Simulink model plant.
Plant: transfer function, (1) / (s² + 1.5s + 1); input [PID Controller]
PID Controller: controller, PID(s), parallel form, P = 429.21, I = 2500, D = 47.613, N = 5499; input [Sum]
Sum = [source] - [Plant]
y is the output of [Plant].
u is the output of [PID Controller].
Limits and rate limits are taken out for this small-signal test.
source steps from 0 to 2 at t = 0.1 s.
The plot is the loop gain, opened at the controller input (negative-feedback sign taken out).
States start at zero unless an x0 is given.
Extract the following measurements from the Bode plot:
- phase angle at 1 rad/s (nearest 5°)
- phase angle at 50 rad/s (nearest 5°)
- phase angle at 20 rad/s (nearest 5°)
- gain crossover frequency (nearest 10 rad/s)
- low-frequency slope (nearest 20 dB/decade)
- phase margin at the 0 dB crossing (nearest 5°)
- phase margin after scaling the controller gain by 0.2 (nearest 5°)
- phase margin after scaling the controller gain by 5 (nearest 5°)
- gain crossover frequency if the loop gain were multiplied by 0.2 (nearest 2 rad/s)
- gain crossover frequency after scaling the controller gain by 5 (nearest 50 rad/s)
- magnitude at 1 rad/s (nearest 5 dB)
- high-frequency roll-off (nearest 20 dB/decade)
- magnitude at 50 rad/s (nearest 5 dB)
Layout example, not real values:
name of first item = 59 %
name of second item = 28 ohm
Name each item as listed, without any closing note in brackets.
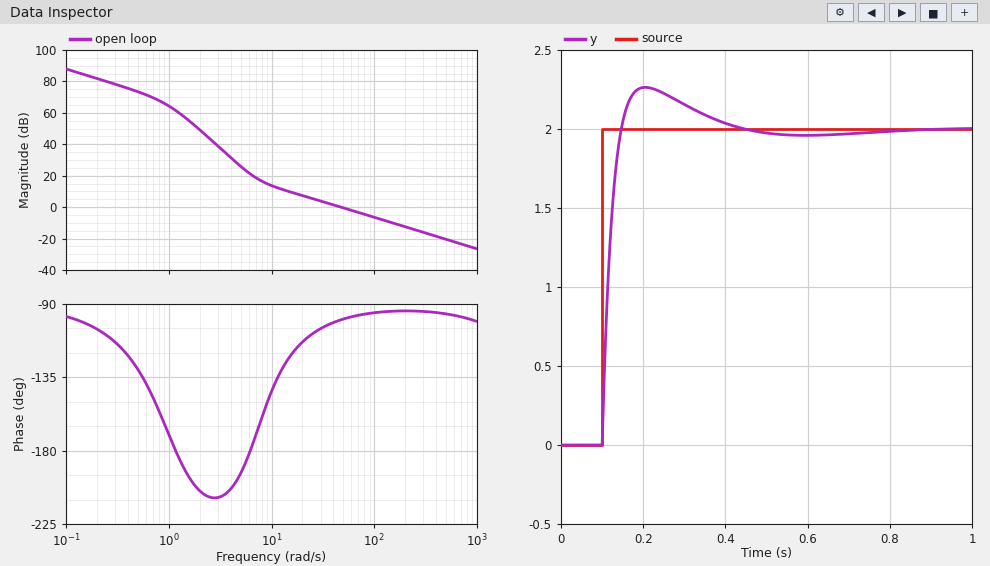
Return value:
phase angle at 1 rad/s = -170°
phase angle at 50 rad/s = -100°
phase angle at 20 rad/s = -115°
gain crossover frequency = 50 rad/s
low-frequency slope = -20 dB/decade
phase margin at the 0 dB crossing = 80°
phase margin after scaling the controller gain by 0.2 = 35°
phase margin after scaling the controller gain by 5 = 85°
gain crossover frequency if the loop gain were multiplied by 0.2 = 10 rad/s
gain crossover frequency after scaling the controller gain by 5 = 250 rad/s
magnitude at 1 rad/s = 65 dB
high-frequency roll-off = -20 dB/decade
magnitude at 50 rad/s = 0 dB
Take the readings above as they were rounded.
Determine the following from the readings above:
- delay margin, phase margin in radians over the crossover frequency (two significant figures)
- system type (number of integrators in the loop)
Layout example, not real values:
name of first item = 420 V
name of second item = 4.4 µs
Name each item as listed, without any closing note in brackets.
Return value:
delay margin, phase margin in radians over the crossover frequency = 0.028 s
system type = 1
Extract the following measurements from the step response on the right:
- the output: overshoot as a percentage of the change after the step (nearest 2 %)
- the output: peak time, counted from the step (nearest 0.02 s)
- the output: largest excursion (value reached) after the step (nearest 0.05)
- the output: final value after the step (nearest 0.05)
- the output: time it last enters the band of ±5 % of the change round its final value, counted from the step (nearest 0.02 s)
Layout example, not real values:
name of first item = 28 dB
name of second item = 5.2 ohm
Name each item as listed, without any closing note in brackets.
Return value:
the output: overshoot as a percentage of the change after the step = 14 %
the output: peak time, counted from the step = 0.10 s
the output: largest excursion (value reached) after the step = 2.25
the output: final value after the step = 2.00
the output: time it last enters the band of ±5 % of the change round its final value, counted from the step = 0.24 s
